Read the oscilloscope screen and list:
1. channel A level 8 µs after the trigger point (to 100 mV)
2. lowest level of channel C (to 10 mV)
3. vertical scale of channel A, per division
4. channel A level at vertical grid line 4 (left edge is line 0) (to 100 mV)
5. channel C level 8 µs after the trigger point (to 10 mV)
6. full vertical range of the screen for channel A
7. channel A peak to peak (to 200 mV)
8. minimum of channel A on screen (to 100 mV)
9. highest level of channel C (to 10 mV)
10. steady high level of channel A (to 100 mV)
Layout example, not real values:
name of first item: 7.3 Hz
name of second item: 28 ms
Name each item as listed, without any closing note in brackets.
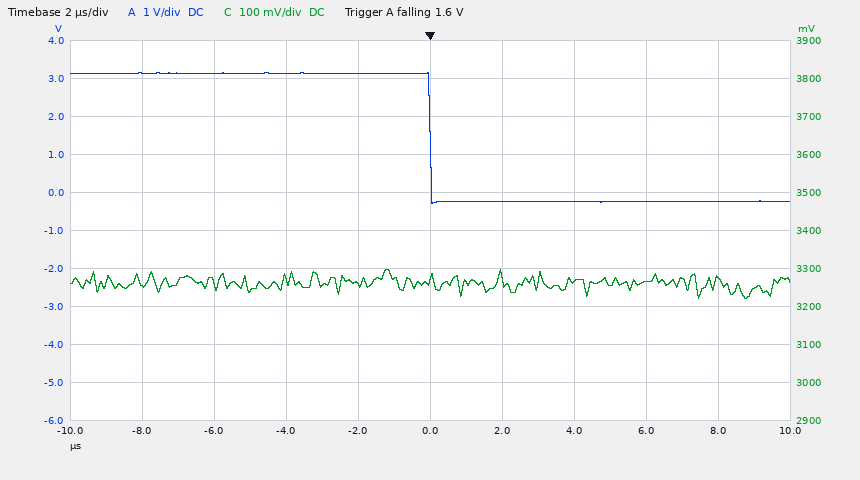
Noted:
channel A level 8 µs after the trigger point: -200 mV
lowest level of channel C: 3.22 V
vertical scale of channel A, per division: 1 V
channel A level at vertical grid line 4 (left edge is line 0): 3.1 V
channel C level 8 µs after the trigger point: 3.27 V
full vertical range of the screen for channel A: 10 V
channel A peak to peak: 3.4 V
minimum of channel A on screen: -300 mV
highest level of channel C: 3.30 V
steady high level of channel A: 3.1 V
